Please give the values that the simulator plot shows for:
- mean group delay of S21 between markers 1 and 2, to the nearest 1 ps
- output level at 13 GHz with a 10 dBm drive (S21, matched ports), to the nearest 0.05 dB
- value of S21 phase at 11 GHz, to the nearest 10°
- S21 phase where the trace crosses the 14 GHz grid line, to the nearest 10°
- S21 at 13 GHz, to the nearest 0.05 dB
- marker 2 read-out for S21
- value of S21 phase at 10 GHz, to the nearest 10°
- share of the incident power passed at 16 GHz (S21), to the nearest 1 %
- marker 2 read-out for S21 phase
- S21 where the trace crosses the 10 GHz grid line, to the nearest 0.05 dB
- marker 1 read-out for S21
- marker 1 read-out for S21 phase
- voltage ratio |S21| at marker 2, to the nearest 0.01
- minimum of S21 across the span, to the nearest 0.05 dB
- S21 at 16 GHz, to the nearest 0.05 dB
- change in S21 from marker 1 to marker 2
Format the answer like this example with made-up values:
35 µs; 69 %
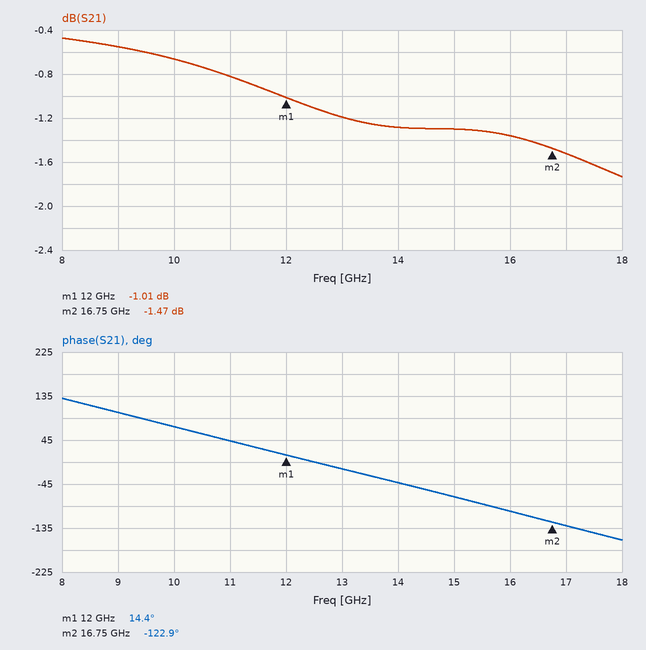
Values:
80 ps; 8.80 dBm; 40°; -40°; -1.20 dB; -1.47 dB; 70°; 73 %; -122.9°; -0.65 dB; -1.01 dB; 14.4°; 0.84; -1.75 dB; -1.35 dB; -0.46 dB
